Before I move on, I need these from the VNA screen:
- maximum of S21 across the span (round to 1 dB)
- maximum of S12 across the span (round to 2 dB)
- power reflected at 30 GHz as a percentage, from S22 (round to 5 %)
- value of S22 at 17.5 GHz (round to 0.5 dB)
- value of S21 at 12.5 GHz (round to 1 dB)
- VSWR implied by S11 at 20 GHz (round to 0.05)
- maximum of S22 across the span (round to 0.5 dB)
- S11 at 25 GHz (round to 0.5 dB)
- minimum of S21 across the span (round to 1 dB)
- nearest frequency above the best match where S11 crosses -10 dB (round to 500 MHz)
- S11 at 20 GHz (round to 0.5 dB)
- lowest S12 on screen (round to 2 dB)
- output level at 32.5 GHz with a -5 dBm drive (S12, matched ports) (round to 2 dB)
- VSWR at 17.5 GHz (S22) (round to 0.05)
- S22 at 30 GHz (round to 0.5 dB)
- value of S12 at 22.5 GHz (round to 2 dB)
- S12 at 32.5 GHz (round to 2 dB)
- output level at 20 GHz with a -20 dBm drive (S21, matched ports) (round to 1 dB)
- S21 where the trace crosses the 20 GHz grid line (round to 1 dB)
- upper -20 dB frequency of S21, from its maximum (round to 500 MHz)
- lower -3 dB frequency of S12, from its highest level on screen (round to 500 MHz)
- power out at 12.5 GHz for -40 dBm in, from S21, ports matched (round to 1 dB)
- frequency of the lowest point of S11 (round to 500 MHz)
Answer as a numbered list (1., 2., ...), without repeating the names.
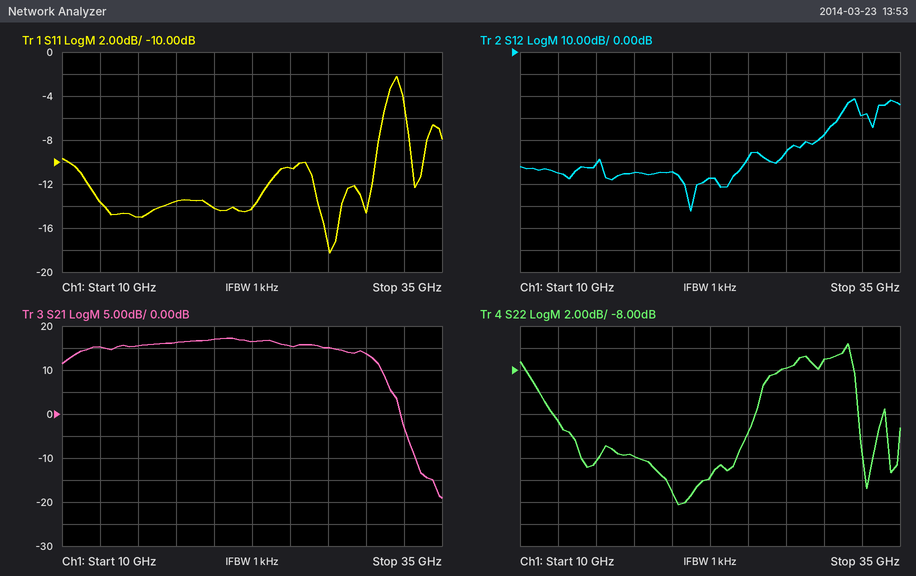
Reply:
1. 17 dB
2. -22 dB
3. 20 %
4. -16.0 dB
5. 15 dB
6. 1.50
7. -5.5 dB
8. -10.5 dB
9. -19 dB
10. 30.5 GHz
11. -14.0 dB
12. -72 dB
13. -34 dBm
14. 1.40
15. -7.0 dB
16. -58 dB
17. -28 dB
18. -3 dBm
19. 17 dB
20. 32.5 GHz
21. 31.5 GHz
22. -25 dBm
23. 27.5 GHz
